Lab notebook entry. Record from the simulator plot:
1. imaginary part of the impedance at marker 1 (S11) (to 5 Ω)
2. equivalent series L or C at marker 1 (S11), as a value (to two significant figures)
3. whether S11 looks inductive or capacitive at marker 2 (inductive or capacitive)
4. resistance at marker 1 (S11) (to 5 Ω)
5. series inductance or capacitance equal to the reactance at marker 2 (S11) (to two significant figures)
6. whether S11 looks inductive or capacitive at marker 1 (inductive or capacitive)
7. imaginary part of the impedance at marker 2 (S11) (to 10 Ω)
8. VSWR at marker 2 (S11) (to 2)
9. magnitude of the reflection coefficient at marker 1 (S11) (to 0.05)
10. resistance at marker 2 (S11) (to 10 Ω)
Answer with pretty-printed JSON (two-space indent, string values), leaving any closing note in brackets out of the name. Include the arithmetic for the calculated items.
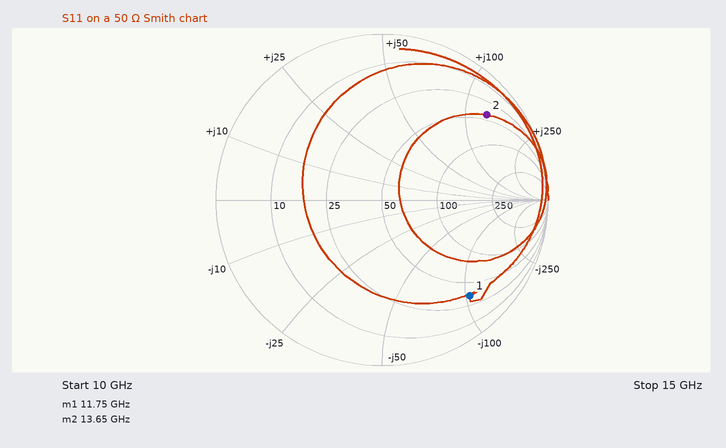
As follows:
{
  "imaginary part of the impedance at marker 1 (S11)": "-105 Ω",
  "equivalent series L or C at marker 1 (S11), as a value": "C = 1/(2π × 11.75 GHz × 105 Ω) ≈ 129 fF, so 130 fF to two significant figures",
  "whether S11 looks inductive or capacitive at marker 2": "inductive",
  "resistance at marker 1 (S11)": "35 Ω",
  "series inductance or capacitance equal to the reactance at marker 2 (S11)": "L = 130 Ω/(2π × 13.65 GHz) ≈ 1.5 nH",
  "whether S11 looks inductive or capacitive at marker 1": "capacitive",
  "imaginary part of the impedance at marker 2 (S11)": "+130 Ω",
  "VSWR at marker 2 (S11)": "10",
  "magnitude of the reflection coefficient at marker 1 (S11)": "0.80",
  "resistance at marker 2 (S11)": "40 Ω"
}
